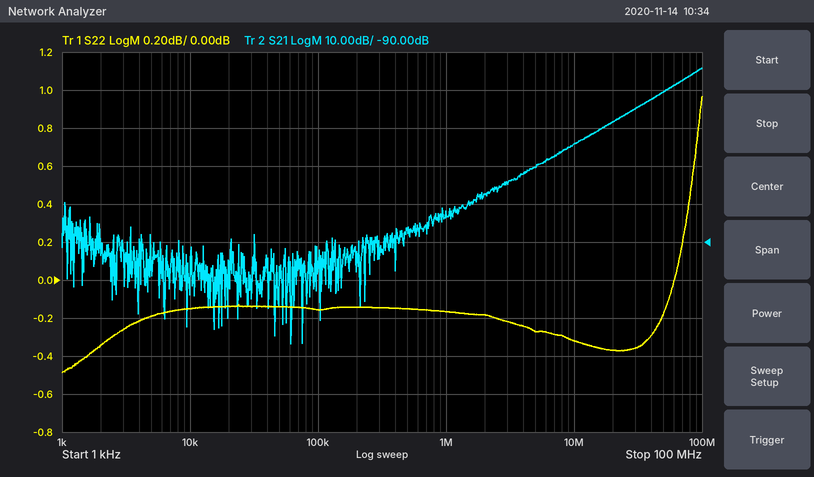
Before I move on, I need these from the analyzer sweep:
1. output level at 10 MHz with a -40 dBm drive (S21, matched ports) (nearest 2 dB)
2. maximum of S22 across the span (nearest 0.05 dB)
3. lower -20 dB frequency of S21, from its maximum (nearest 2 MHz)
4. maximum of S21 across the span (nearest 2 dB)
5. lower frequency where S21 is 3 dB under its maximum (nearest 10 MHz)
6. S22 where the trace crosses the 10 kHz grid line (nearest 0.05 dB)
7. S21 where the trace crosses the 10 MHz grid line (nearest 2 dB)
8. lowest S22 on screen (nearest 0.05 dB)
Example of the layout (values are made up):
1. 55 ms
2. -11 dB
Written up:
1. -104 dBm
2. 0.95 dB
3. 10 MHz
4. -44 dB
5. 70 MHz
6. -0.15 dB
7. -64 dB
8. -0.50 dB
